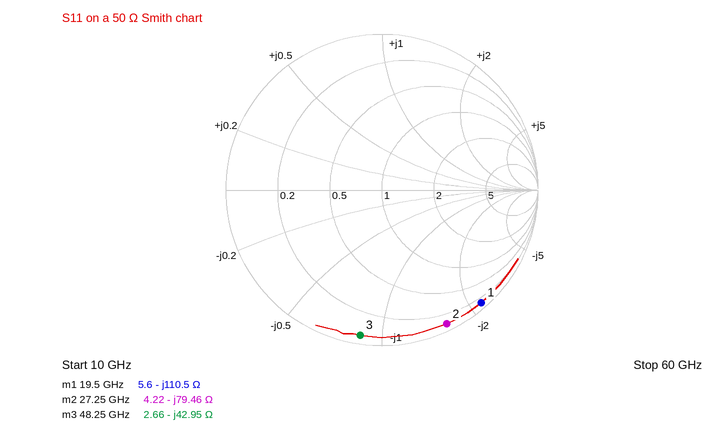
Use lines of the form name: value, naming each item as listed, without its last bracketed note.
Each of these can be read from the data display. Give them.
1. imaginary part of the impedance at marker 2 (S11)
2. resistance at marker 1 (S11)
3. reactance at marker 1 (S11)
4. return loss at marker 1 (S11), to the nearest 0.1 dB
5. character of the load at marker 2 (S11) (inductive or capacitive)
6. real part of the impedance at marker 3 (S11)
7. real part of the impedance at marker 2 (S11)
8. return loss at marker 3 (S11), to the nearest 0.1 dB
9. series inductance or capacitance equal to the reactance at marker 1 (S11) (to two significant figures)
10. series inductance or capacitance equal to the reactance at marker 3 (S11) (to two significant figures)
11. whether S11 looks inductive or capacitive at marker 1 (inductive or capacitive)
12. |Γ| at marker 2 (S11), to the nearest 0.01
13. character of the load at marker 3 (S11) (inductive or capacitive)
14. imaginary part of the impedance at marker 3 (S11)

imaginary part of the impedance at marker 2: -79.46 Ω
resistance at marker 1: 5.6 Ω
reactance at marker 1: -110.5 Ω
return loss at marker 1 (S11), to the nearest 0.1 dB: 0.3 dB
character of the load at marker 2 (S11): capacitive
real part of the impedance at marker 3: 2.66 Ω
real part of the impedance at marker 2: 4.22 Ω
return loss at marker 3 (S11), to the nearest 0.1 dB: 0.5 dB
series inductance or capacitance equal to the reactance at marker 1 (S11): 74 fF
series inductance or capacitance equal to the reactance at marker 3 (S11): 77 fF
whether S11 looks inductive or capacitive at marker 1: capacitive
|Γ| at marker 2 (S11), to the nearest 0.01: 0.95
character of the load at marker 3 (S11): capacitive
imaginary part of the impedance at marker 3: -42.95 Ω
